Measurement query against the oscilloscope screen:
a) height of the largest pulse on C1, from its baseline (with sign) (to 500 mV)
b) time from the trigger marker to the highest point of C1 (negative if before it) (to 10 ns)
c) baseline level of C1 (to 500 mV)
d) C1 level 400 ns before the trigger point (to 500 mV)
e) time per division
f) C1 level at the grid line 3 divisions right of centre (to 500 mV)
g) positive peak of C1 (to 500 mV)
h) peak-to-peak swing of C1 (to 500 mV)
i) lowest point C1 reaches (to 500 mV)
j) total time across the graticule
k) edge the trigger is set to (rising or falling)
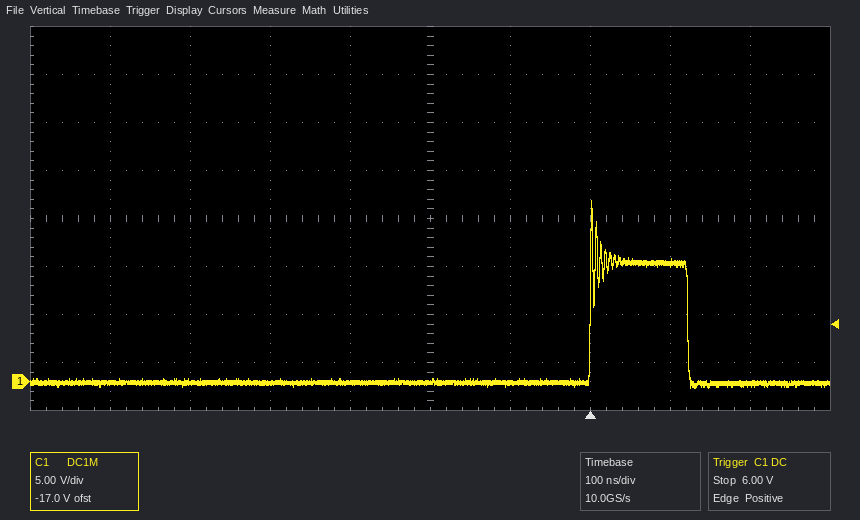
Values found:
+19.0 V
0 ns
0.0 V
0.0 V
100 ns
12.5 V
19.0 V
19.5 V
-500 mV
1 µs
rising
